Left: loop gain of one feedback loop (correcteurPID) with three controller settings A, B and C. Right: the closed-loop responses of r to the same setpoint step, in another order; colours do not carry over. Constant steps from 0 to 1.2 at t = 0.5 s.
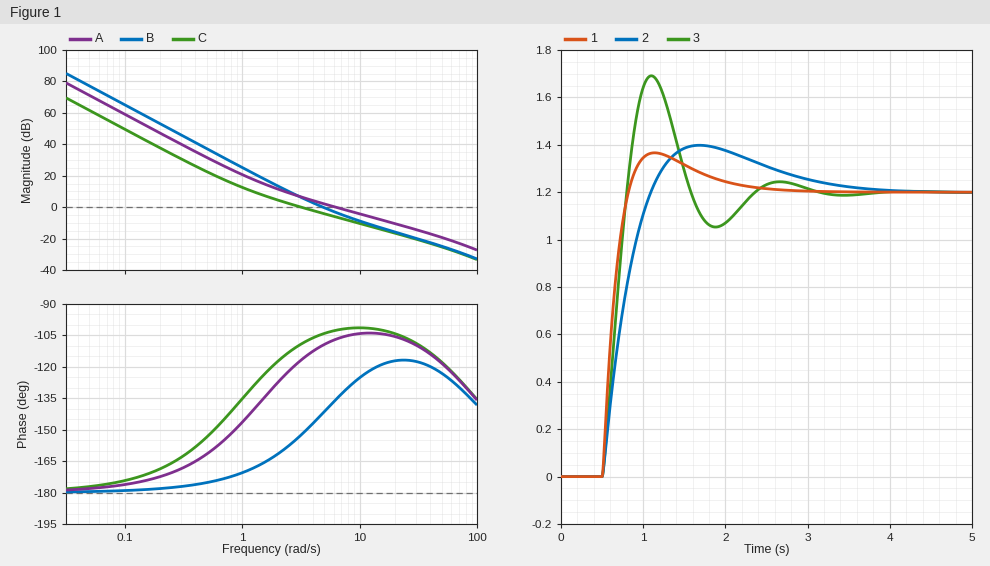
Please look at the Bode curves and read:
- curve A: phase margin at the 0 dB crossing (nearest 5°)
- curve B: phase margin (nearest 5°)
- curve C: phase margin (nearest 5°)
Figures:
75°
40°
70°
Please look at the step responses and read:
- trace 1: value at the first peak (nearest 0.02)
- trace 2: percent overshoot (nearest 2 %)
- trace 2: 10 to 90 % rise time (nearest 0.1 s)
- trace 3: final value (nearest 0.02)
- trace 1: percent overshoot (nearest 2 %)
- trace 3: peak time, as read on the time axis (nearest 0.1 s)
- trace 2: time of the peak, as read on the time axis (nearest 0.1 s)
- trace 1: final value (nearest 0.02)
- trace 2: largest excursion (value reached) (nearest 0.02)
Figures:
1.36
16 %
0.4 s
1.20
14 %
1.1 s
1.7 s
1.20
1.40
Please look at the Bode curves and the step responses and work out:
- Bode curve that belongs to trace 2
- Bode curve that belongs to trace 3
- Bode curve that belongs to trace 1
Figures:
C
B
A
